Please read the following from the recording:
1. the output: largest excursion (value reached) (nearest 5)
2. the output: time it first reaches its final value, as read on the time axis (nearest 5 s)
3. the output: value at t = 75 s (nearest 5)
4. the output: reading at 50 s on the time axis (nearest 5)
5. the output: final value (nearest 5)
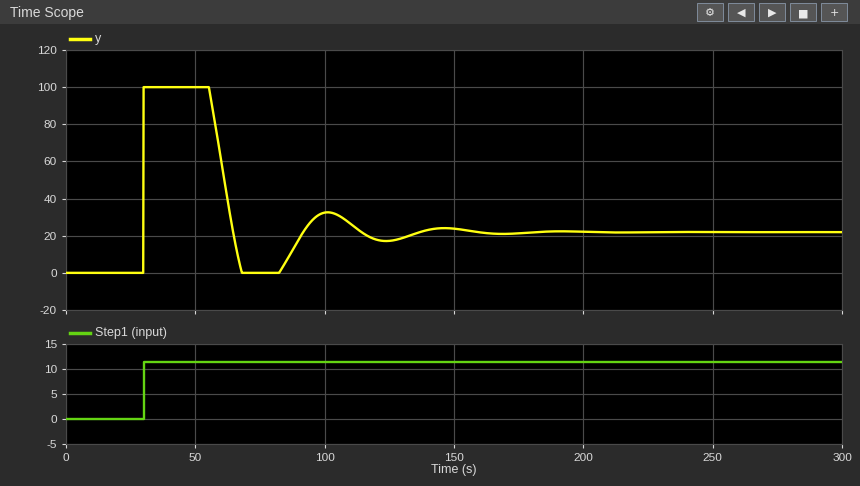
100
30 s
0
100
20
